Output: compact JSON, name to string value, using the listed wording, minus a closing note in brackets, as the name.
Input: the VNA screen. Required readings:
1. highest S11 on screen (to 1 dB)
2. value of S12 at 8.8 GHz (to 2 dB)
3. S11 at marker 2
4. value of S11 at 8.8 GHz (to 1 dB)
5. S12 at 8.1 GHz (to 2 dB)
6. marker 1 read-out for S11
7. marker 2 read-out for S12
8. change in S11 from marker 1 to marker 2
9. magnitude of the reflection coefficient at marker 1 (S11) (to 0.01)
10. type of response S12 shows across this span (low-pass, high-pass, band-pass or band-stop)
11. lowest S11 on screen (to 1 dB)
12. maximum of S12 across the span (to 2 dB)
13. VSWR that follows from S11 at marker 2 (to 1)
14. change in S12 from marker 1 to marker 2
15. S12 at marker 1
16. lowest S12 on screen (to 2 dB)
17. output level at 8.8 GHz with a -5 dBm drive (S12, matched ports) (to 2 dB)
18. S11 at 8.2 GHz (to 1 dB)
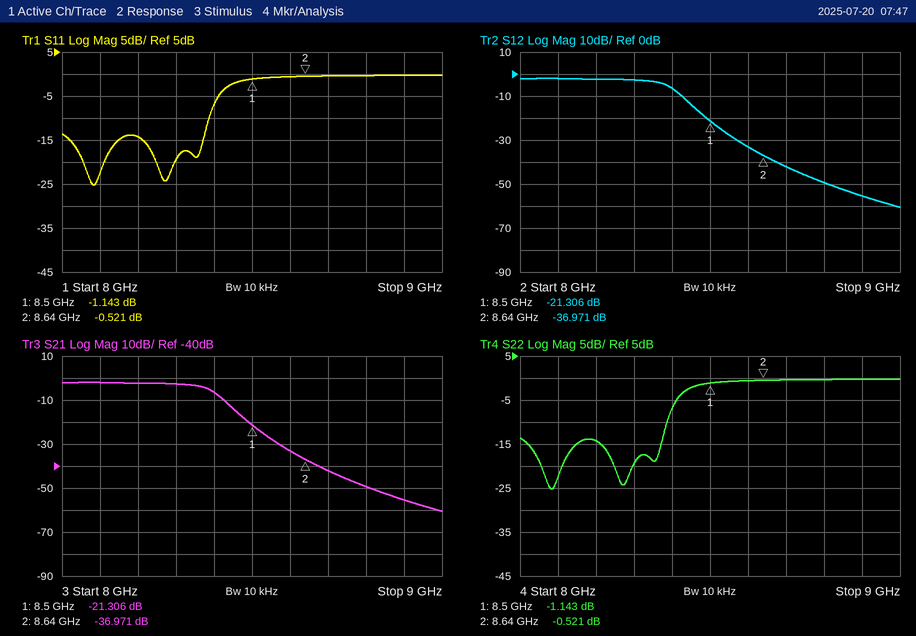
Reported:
{"highest S11 on screen": "0 dB", "value of S12 at 8.8 GHz": "-50 dB", "S11 at marker 2": "-0.521 dB", "value of S11 at 8.8 GHz": "0 dB", "S12 at 8.1 GHz": "-2 dB", "marker 1 read-out for S11": "-1.143 dB", "marker 2 read-out for S12": "-36.971 dB", "change in S11 from marker 1 to marker 2": "0.622 dB", "magnitude of the reflection coefficient at marker 1 (S11)": "0.88", "type of response S12 shows across this span": "low-pass", "lowest S11 on screen": "-25 dB", "maximum of S12 across the span": "-2 dB", "VSWR that follows from S11 at marker 2": "33", "change in S12 from marker 1 to marker 2": "-15.665 dB", "S12 at marker 1": "-21.306 dB", "lowest S12 on screen": "-60 dB", "output level at 8.8 GHz with a -5 dBm drive (S12, matched ports)": "-54 dBm", "S11 at 8.2 GHz": "-14 dB"}
